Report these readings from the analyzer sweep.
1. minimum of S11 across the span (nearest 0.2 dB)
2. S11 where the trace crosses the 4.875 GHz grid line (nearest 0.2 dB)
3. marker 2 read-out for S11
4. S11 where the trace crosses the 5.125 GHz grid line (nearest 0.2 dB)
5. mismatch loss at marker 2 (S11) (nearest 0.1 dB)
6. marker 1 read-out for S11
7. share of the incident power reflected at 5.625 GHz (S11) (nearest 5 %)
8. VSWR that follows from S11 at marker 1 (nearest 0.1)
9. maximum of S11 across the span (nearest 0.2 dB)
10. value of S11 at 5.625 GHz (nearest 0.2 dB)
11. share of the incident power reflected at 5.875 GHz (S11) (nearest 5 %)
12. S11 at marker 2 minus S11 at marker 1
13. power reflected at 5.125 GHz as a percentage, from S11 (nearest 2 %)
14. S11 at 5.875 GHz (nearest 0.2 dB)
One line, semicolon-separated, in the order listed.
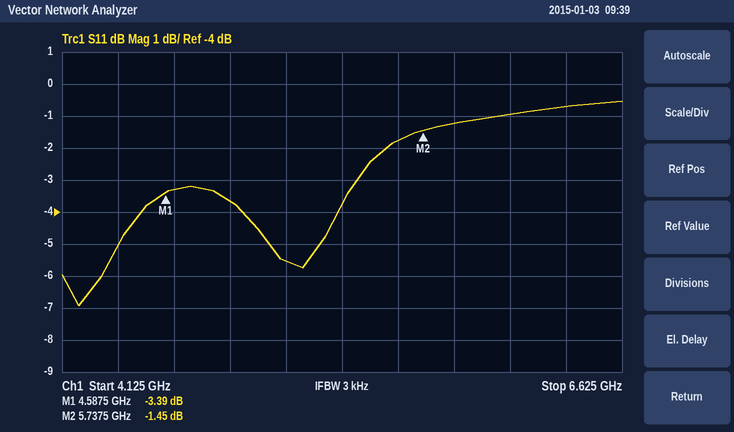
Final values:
-7.0 dB; -3.6 dB; -1.45 dB; -5.6 dB; 5.5 dB; -3.39 dB; 65 %; 5.2; -0.6 dB; -1.8 dB; 75 %; 1.94 dB; 28 %; -1.2 dB
